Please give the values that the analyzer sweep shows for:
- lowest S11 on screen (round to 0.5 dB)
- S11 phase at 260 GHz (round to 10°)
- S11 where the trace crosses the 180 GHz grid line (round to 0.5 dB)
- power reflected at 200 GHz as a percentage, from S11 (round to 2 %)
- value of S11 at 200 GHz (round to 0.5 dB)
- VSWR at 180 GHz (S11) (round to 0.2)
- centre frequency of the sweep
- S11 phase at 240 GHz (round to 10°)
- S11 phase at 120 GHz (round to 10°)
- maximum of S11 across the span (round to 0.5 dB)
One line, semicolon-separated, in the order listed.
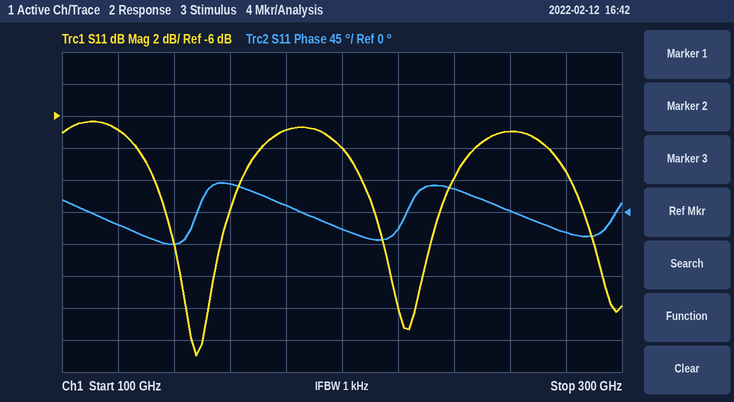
-21.0 dB; 0°; -7.0 dB; 16 %; -8.0 dB; 2.6; 200 GHz; 30°; -20°; -6.5 dB
